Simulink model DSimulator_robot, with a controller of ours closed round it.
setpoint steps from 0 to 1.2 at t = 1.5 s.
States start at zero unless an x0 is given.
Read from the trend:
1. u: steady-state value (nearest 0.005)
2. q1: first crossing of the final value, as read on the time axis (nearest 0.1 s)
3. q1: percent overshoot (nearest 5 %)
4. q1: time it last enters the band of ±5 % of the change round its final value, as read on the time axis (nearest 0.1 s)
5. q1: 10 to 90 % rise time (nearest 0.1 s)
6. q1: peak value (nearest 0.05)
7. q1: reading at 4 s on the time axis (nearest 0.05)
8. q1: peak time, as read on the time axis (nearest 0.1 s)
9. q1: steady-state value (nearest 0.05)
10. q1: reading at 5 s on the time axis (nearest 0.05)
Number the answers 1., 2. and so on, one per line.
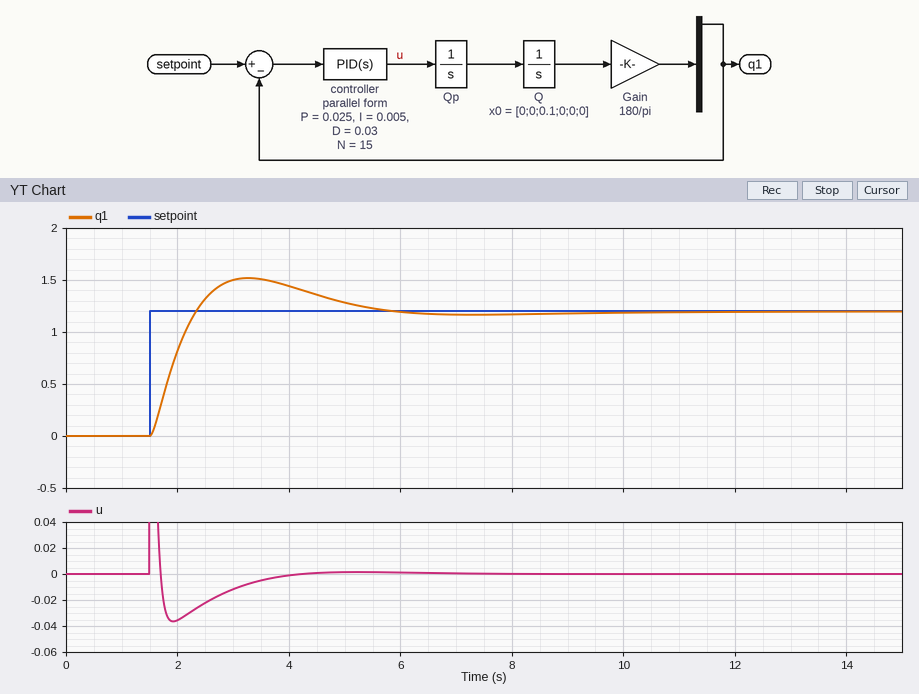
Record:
1. 0.000
2. 2.3 s
3. 25 %
4. 5.2 s
5. 0.6 s
6. 1.50
7. 1.45
8. 3.3 s
9. 1.20
10. 1.30
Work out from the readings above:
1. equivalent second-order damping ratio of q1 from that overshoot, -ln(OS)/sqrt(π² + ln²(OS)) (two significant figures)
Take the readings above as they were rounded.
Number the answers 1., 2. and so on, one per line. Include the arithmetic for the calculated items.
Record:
1. ln(0.25) = -1.386; 1.386 / sqrt(9.870 + 1.922) = 0.40
